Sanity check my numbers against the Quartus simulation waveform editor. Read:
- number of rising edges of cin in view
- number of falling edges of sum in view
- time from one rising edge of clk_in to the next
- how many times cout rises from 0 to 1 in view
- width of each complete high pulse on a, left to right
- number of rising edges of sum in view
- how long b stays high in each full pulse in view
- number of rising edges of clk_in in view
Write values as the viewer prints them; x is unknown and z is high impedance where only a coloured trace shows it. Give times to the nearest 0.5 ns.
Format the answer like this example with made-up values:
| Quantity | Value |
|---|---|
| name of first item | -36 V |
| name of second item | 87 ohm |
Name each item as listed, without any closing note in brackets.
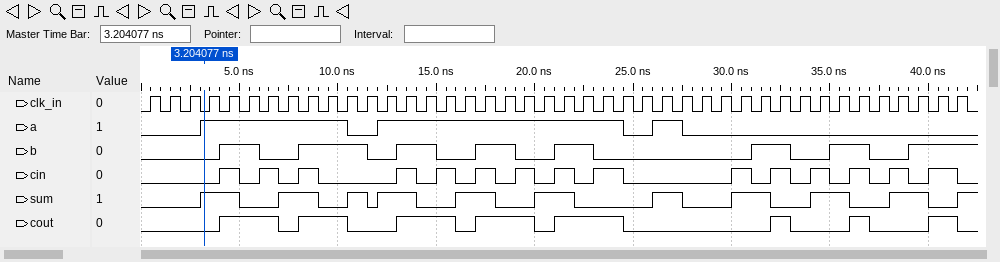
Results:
| Quantity | Value |
|---|---|
| number of rising edges of cin in view | 15 |
| number of falling edges of sum in view | 10 |
| time from one rising edge of clk_in to the next | 1 ns |
| how many times cout rises from 0 to 1 in view | 8 |
| width of each complete high pulse on a, left to right | 7.5 ns, 12.5 ns, 1.5 ns |
| number of rising edges of sum in view | 11 |
| how long b stays high in each full pulse in view | 2 ns, 3.5 ns, 2 ns, 2 ns, 2 ns, 2 ns, 2 ns |
| number of rising edges of clk_in in view | 42 |
